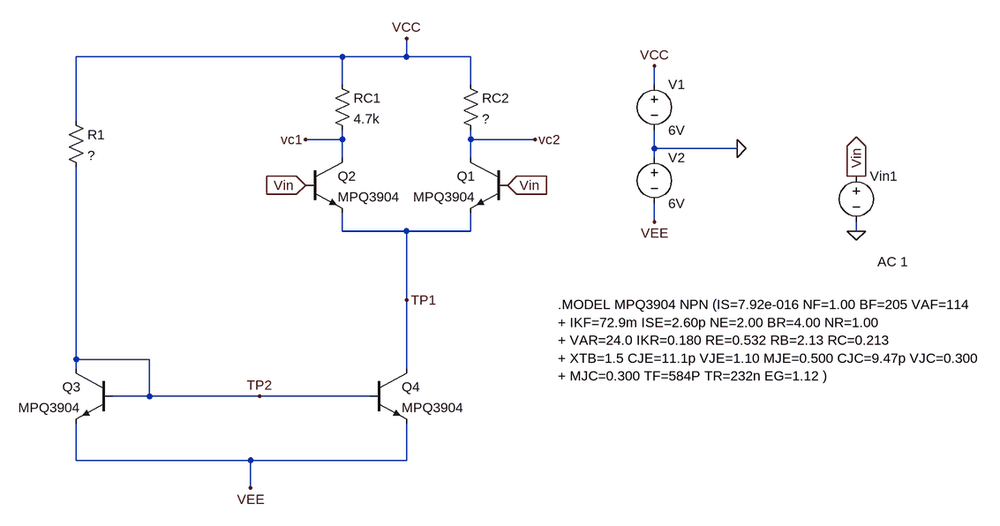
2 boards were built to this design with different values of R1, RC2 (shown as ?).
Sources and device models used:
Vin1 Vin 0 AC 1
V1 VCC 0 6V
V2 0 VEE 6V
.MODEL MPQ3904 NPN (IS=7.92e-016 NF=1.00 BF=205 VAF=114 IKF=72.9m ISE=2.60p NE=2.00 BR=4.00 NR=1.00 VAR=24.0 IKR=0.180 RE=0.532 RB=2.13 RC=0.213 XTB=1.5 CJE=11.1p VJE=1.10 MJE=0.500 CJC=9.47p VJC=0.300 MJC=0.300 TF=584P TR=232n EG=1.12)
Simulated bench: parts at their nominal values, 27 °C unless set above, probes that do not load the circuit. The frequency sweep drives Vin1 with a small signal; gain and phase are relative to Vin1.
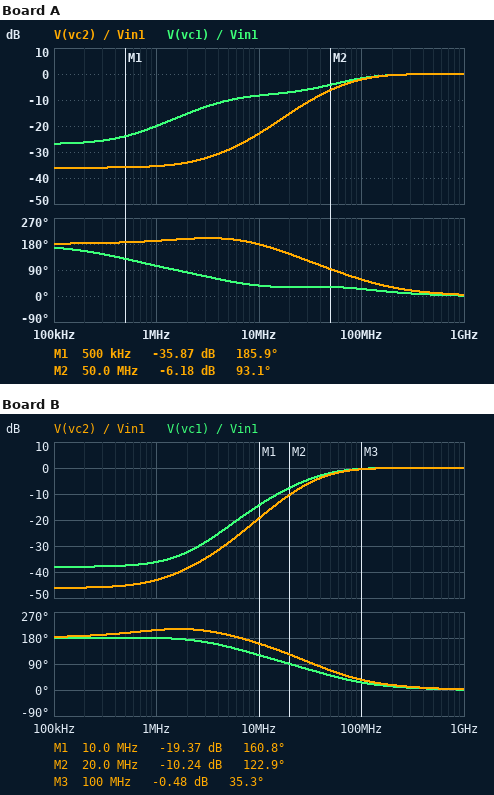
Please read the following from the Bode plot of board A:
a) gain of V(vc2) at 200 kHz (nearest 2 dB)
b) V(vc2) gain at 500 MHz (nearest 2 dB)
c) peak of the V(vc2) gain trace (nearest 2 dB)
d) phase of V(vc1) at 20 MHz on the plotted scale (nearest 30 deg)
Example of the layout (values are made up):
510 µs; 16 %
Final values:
-36 dB; 0 dB; 0 dB; 30 deg
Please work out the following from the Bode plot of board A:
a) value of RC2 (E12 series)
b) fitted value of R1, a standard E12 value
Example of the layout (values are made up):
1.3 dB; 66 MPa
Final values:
1.5 kΩ; 4.7 kΩ
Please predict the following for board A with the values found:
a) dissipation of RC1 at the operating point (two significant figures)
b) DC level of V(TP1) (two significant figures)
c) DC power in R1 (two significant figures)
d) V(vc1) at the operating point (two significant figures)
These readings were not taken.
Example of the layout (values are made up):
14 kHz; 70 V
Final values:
6.7 mW; -730 mV; 27 mW; 370 mV
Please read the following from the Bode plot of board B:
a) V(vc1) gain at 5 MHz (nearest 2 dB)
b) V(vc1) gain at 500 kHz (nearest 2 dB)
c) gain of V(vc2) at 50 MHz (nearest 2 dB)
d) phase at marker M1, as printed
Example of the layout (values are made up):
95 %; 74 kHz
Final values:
-22 dB; -38 dB; -2 dB; 160.8 deg
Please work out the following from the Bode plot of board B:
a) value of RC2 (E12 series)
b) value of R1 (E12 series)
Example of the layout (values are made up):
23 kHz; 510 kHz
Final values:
1.8 kΩ; 18 kΩ
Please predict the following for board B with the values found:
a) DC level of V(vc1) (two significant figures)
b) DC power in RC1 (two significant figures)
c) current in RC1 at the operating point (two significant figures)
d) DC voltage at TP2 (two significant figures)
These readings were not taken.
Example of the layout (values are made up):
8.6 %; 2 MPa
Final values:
4.5 V; 470 µW; 320 µA; -5.3 V
